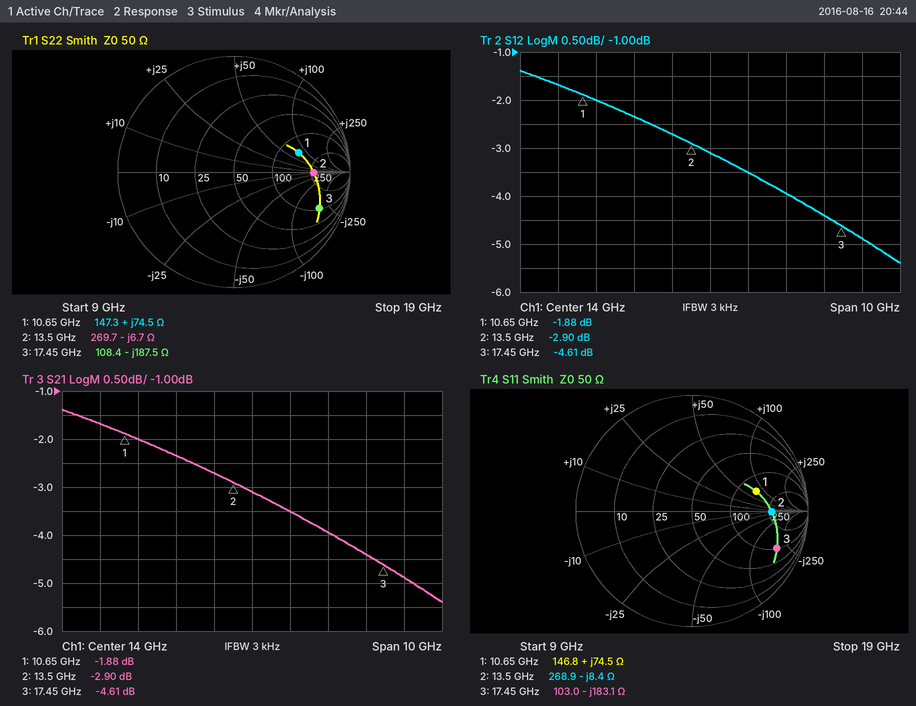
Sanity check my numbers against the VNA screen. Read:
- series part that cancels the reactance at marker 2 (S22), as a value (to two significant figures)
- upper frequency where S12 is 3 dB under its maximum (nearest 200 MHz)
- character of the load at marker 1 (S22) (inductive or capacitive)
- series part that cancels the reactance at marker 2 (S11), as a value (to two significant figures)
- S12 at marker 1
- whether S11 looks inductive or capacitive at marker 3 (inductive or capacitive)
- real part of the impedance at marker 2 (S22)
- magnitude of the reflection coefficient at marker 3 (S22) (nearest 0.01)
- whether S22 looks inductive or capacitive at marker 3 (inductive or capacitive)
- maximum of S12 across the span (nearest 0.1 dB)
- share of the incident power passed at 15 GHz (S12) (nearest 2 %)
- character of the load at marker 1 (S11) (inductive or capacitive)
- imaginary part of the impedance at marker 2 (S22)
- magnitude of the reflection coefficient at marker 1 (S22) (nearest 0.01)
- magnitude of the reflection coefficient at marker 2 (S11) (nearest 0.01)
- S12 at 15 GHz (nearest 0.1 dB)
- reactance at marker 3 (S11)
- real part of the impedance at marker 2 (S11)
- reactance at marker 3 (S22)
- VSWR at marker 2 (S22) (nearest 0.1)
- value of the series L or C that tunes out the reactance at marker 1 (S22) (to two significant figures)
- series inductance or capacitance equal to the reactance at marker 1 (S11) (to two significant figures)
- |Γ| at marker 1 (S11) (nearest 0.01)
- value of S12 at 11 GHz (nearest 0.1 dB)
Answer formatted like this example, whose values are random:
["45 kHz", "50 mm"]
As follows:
["79 pH", "17.0 GHz", "inductive", "99 pH", "-1.88 dB", "capacitive", "269.7 Ω", "0.80", "capacitive", "-1.4 dB", "44 %", "inductive", "-6.7 Ω", "0.58", "0.69", "-3.5 dB", "-183.1 Ω", "268.9 Ω", "-187.5 Ω", "5.4", "200 fF", "1.1 nH", "0.58", "-2.0 dB"]
